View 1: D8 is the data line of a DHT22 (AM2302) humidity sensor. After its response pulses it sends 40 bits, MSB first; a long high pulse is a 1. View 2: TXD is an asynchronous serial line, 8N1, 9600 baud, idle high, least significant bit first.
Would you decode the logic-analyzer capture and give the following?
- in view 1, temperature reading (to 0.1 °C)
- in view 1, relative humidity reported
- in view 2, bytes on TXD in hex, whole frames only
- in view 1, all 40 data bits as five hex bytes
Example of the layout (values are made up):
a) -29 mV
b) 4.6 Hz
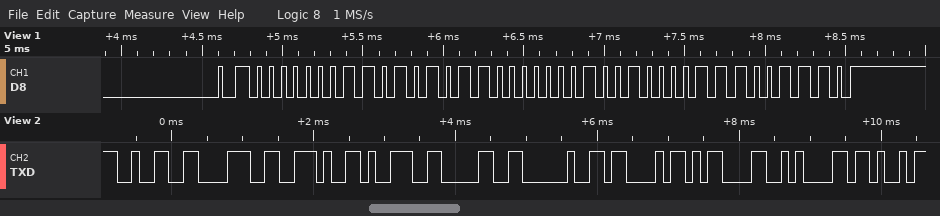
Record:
a) 28.9 °C
b) 42.7 %
c) 0x32 0x38 0x2E 0x39 0x30 0x20 0x43 0x0D 0x0A 0x4B
d) 01 AB 01 21 CE
